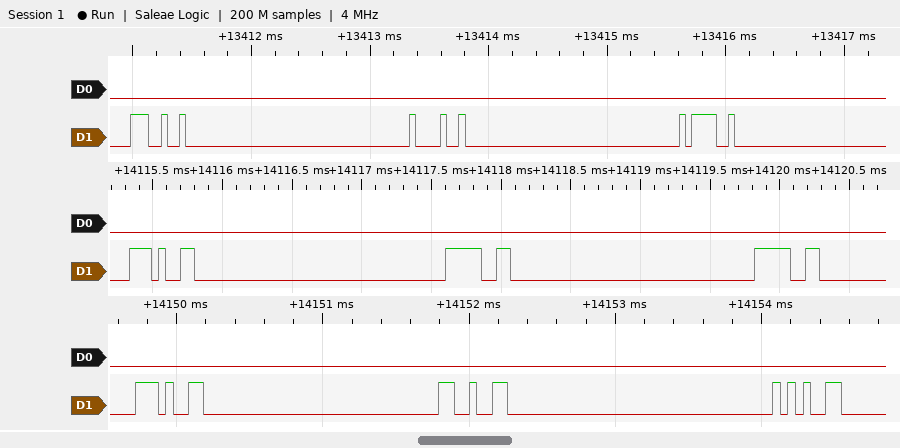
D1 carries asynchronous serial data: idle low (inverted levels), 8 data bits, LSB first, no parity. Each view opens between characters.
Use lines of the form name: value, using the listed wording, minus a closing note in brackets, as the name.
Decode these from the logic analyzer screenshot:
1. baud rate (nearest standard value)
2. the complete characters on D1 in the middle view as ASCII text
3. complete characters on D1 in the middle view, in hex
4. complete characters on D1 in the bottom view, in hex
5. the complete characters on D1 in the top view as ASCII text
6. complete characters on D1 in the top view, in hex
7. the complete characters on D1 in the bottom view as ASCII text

baud rate: 19200 baud
the complete characters on D1 in the middle view as ASCII text: "400"
complete characters on D1 in the middle view, in hex: 34, 30, 30
complete characters on D1 in the bottom view, in hex: 34, 36, 35
the complete characters on D1 in the top view as ASCII text: "loa"
complete characters on D1 in the top view, in hex: 6C, 6F, 61
the complete characters on D1 in the bottom view as ASCII text: "465"
